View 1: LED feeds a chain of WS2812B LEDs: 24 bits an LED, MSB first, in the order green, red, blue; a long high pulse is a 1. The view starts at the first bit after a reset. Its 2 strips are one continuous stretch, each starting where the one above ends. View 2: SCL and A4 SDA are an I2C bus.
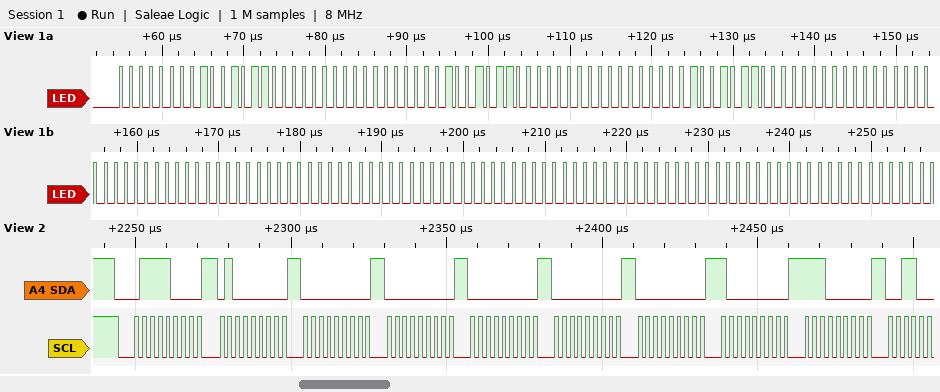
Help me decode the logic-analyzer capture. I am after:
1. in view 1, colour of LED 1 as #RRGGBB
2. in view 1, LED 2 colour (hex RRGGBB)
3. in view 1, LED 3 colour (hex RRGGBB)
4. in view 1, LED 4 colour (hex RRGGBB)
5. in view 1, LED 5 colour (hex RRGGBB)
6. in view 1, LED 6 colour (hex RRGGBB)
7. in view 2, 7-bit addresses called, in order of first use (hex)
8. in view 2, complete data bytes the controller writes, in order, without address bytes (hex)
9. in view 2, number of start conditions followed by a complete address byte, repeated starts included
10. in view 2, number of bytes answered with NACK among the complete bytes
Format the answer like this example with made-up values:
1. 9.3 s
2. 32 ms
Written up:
1. #960000
2. #960000
3. #960000
4. #000000
5. #000000
6. #000000
7. 0x3C
8. 40 00 00 00 00 00 80 E0
9. 1
10. 0
